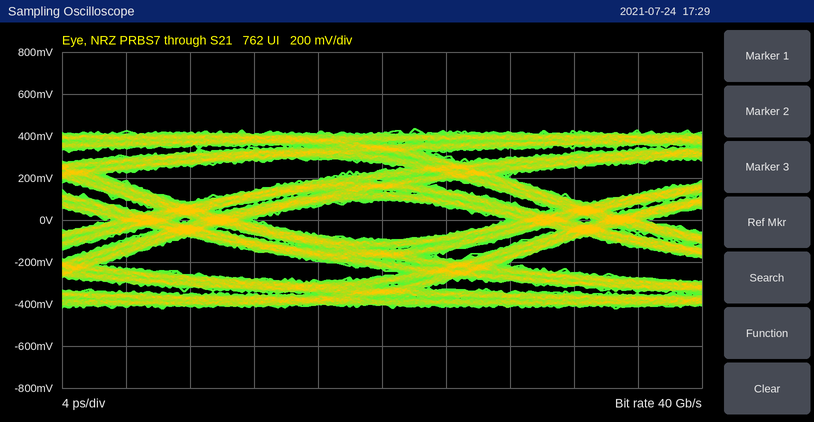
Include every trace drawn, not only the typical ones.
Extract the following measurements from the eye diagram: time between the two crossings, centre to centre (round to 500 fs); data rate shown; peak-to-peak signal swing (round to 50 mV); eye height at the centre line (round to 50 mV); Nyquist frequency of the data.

25.0 ps
40 Gb/s
850 mV
200 mV
20 GHz
